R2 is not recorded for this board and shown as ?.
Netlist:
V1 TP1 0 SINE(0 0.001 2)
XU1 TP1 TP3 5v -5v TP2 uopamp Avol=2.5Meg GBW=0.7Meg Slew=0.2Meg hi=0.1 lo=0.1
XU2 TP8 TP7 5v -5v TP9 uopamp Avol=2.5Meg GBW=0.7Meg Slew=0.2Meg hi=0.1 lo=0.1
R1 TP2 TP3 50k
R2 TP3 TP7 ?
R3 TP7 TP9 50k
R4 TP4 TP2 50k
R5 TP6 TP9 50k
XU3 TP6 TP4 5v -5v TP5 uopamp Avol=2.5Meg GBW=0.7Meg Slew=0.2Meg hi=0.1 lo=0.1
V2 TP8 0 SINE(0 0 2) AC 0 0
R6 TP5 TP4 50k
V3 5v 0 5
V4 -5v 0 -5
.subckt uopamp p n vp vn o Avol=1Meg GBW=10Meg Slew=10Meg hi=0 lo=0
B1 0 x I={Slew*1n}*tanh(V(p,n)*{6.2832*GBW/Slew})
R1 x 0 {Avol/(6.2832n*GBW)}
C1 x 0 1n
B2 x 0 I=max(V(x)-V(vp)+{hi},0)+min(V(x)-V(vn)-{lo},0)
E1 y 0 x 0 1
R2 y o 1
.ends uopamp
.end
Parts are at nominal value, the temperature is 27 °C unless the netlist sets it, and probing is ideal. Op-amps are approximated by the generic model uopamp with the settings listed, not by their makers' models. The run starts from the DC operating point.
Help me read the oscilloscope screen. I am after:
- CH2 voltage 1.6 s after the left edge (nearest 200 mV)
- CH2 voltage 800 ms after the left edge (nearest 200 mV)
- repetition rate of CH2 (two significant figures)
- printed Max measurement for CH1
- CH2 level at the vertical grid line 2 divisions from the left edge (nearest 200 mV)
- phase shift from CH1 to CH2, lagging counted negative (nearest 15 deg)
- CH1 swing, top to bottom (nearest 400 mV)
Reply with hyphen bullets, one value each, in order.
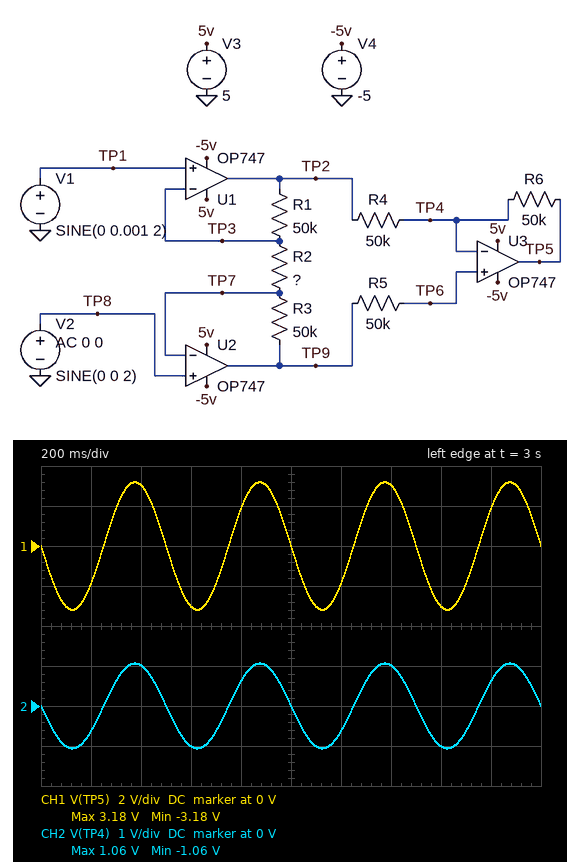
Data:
- -1.0 V
- 600 mV
- 2.0 Hz
- 3.18 V
- 1.0 V
- 0 deg
- 6.4 V
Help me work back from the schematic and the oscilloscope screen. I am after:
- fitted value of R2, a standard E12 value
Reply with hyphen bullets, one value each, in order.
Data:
- 47 Ω
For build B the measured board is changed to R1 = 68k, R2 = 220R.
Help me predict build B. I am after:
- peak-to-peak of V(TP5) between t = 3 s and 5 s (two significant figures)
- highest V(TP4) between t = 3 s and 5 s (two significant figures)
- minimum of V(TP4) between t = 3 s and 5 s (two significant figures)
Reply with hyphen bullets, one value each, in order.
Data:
- 1.5 V
- 230 mV
- -230 mV
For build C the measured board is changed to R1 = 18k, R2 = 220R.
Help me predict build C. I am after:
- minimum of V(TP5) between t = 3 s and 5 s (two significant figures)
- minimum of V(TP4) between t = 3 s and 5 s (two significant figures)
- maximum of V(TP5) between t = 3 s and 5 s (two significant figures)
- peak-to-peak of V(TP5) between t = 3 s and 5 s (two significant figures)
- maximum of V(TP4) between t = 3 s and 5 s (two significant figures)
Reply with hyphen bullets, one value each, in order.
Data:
- -540 mV
- -230 mV
- 540 mV
- 1.1 V
- 230 mV
